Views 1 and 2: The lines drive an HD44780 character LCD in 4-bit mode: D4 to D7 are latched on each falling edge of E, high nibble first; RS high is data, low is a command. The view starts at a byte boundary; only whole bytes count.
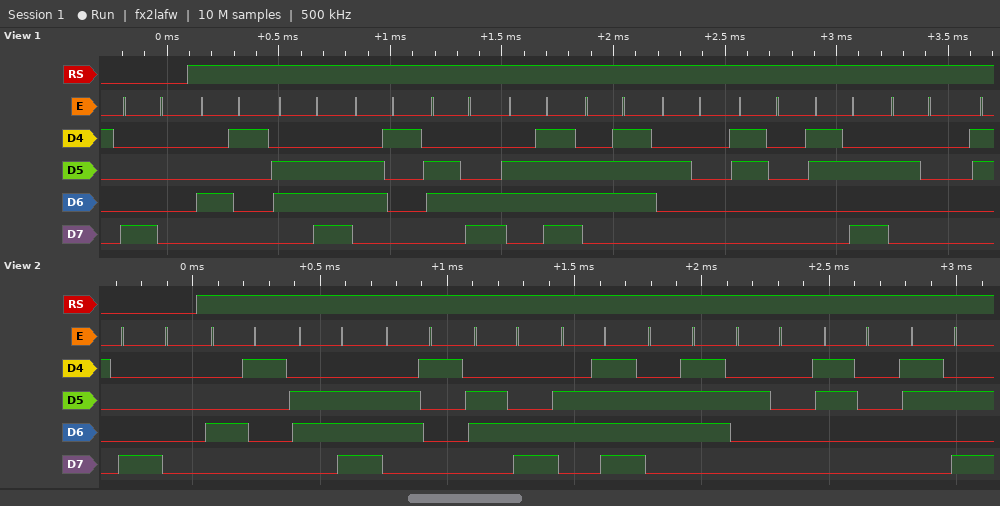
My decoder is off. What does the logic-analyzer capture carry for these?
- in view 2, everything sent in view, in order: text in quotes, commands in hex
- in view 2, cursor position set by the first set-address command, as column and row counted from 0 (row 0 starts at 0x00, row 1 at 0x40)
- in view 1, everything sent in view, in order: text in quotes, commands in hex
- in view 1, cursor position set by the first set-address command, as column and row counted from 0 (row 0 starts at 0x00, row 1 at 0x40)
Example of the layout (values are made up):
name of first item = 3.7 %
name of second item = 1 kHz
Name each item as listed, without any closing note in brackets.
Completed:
in view 2, everything sent in view, in order: text in quotes, commands in hex = 0x80 "Analog 0:"
in view 2, cursor position set by the first set-address command, as column and row counted from 0 = column 0, row 0
in view 1, everything sent in view, in order: text in quotes, commands in hex = 0x80 "Analog 0: "
in view 1, cursor position set by the first set-address command, as column and row counted from 0 = column 0, row 0
